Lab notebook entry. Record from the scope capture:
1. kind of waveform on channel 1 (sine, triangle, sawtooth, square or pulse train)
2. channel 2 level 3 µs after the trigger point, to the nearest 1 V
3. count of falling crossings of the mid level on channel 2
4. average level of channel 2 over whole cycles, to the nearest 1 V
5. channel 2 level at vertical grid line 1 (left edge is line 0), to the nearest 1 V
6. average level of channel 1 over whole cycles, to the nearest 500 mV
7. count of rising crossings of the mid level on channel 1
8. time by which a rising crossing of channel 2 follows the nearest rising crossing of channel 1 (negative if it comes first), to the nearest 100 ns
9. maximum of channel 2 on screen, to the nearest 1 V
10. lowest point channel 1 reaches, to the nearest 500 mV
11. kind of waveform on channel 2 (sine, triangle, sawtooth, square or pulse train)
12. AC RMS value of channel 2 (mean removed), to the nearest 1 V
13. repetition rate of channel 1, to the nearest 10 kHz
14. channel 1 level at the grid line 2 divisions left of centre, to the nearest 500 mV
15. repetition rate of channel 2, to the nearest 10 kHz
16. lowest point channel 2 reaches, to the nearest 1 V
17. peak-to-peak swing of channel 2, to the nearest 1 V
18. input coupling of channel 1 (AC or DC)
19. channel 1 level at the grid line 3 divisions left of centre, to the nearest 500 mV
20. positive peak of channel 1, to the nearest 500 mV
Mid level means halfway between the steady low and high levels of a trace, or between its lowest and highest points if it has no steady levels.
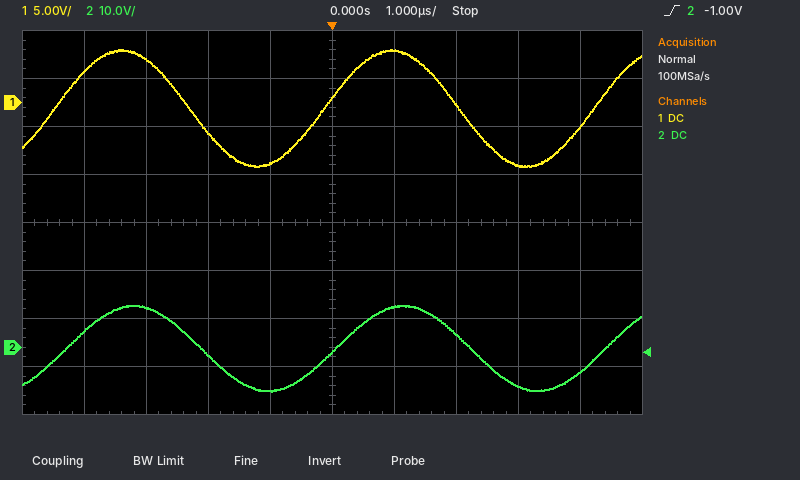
sine
-8 V
2
0 V
3 V
-500 mV
3
+200 ns
9 V
-6.5 V
sine
6 V
230 kHz
-3.0 V
230 kHz
-9 V
18 V
DC
4.5 V
5.5 V
